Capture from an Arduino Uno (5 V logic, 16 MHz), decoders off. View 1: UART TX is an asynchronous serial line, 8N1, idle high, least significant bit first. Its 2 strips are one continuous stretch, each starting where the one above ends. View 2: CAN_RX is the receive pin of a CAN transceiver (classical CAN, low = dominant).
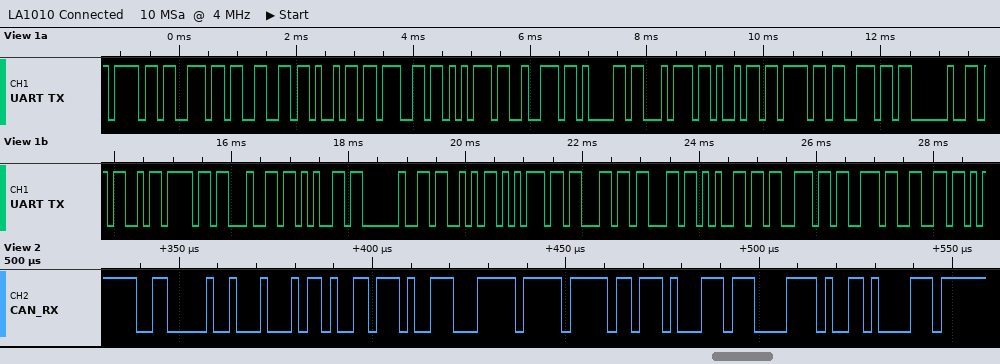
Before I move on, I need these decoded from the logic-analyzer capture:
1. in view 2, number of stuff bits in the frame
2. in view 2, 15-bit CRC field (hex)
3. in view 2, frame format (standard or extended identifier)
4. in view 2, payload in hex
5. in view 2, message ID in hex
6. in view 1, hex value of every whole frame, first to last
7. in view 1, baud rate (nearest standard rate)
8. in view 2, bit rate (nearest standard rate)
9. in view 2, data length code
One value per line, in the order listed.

4
0x5343
standard
B4 DD 38 FF FF BA 3B 87
0x301
6F 6E 66 69 67 75 72 61 74 69 6F 6E 20 4D 6F 64 65 20 53 75 63 63 65 73 73 66
9600 baud
500 kbit/s
8
